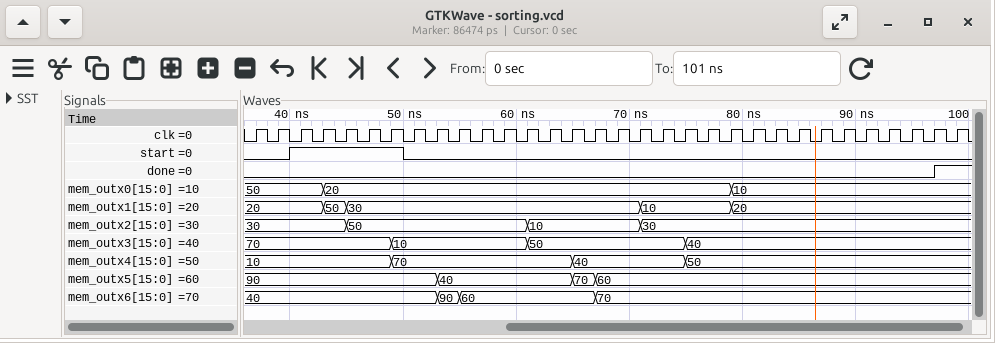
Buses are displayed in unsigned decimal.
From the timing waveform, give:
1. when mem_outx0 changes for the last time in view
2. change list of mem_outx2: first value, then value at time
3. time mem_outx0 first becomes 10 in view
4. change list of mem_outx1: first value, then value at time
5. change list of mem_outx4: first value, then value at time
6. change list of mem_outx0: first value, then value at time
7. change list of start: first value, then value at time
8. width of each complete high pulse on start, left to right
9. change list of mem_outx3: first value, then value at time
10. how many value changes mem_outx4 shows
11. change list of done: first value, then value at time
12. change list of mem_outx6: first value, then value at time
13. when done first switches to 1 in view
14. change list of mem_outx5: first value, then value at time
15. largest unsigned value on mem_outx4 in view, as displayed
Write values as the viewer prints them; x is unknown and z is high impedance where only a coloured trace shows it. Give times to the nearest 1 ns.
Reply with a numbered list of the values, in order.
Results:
1. 79 ns
2. 30, 50 at 45 ns, 10 at 61 ns, 30 at 71 ns
3. 79 ns
4. 20, 50 at 43 ns, 30 at 45 ns, 10 at 71 ns, 20 at 79 ns
5. 10, 70 at 49 ns, 40 at 65 ns, 50 at 75 ns
6. 50, 20 at 43 ns, 10 at 79 ns
7. 0, 1 at 40 ns, 0 at 50 ns
8. 10 ns
9. 70, 10 at 49 ns, 50 at 61 ns, 40 at 75 ns
10. 3
11. 0, 1 at 97 ns
12. 40, 90 at 53 ns, 60 at 55 ns, 70 at 67 ns
13. 97 ns
14. 90, 40 at 53 ns, 70 at 65 ns, 60 at 67 ns
15. 70
